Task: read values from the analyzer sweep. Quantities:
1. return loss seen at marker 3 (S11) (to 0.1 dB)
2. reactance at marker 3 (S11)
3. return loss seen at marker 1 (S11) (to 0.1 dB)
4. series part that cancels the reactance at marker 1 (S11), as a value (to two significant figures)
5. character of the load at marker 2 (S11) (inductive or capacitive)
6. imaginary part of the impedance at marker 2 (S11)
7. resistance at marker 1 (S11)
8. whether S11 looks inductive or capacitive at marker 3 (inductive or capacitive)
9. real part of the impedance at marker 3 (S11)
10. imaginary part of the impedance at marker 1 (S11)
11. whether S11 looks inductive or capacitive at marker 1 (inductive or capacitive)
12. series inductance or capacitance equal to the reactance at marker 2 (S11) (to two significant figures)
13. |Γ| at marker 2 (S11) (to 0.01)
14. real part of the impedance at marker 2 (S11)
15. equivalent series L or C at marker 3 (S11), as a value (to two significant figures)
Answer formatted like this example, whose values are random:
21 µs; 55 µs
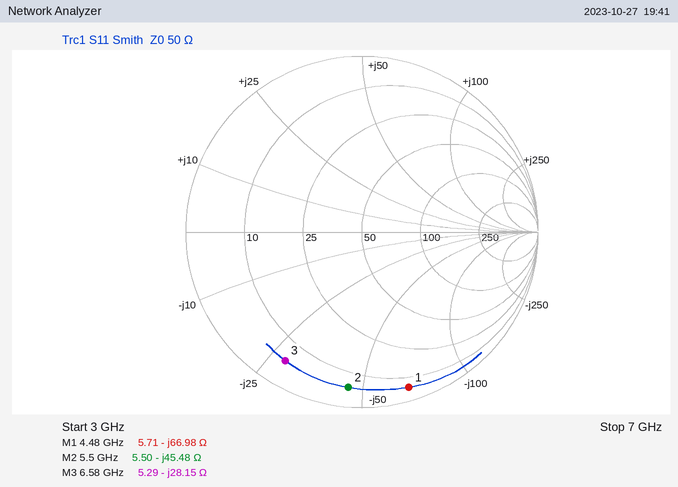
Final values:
1.4 dB; -28.15 Ω; 0.7 dB; 2.4 nH; capacitive; -45.48 Ω; 5.71 Ω; capacitive; 5.29 Ω; -66.98 Ω; capacitive; 640 fF; 0.89; 5.50 Ω; 860 fF
